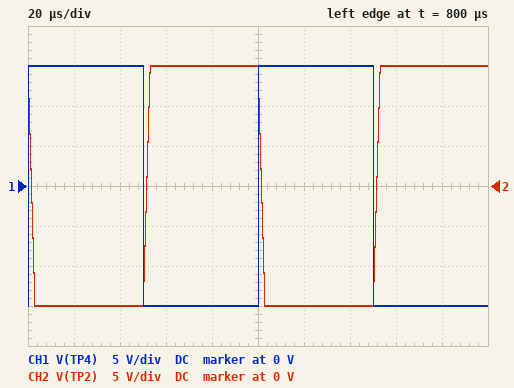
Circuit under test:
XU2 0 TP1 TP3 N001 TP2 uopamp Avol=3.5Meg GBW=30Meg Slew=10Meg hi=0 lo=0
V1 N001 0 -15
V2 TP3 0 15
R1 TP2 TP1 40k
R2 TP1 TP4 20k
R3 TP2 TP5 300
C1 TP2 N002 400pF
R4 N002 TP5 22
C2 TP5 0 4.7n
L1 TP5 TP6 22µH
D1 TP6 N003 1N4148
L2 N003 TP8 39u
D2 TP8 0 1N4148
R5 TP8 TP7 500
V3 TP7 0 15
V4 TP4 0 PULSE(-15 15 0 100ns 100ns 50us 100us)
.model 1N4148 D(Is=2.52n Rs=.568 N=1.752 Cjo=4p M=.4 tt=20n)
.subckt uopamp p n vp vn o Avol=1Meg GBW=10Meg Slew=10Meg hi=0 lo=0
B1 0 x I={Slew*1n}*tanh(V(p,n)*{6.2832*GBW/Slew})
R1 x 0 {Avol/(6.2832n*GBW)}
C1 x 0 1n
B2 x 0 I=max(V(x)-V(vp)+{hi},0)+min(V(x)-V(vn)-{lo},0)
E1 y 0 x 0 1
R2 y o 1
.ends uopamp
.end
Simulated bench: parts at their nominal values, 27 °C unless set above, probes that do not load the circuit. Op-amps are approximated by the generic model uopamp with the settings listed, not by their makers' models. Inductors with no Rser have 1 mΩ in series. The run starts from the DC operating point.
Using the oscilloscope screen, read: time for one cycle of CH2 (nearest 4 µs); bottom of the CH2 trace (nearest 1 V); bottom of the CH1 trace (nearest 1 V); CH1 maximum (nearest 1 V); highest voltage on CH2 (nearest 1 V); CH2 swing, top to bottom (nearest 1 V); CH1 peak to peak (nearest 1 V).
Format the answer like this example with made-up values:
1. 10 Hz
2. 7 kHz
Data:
1. 100 µs
2. -15 V
3. -15 V
4. 15 V
5. 15 V
6. 30 V
7. 30 V
